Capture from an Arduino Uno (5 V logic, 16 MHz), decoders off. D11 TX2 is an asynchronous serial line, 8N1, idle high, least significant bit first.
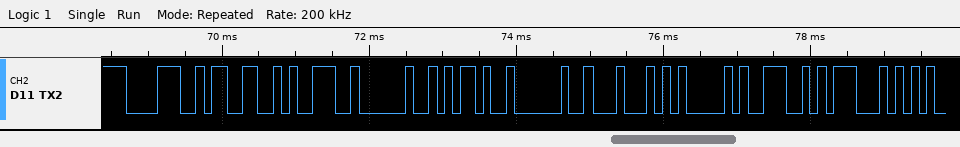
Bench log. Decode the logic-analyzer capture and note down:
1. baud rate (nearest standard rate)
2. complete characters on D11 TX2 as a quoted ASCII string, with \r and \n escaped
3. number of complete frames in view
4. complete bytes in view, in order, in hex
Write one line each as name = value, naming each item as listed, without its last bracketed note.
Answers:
baud rate = 9600 baud
complete characters on D11 TX2 as a quoted ASCII string, with \r and \n escaped = "839 - DANG"
number of complete frames in view = 10
complete bytes in view, in order, in hex = 38 33 39 20 2D 20 44 41 4E 47
